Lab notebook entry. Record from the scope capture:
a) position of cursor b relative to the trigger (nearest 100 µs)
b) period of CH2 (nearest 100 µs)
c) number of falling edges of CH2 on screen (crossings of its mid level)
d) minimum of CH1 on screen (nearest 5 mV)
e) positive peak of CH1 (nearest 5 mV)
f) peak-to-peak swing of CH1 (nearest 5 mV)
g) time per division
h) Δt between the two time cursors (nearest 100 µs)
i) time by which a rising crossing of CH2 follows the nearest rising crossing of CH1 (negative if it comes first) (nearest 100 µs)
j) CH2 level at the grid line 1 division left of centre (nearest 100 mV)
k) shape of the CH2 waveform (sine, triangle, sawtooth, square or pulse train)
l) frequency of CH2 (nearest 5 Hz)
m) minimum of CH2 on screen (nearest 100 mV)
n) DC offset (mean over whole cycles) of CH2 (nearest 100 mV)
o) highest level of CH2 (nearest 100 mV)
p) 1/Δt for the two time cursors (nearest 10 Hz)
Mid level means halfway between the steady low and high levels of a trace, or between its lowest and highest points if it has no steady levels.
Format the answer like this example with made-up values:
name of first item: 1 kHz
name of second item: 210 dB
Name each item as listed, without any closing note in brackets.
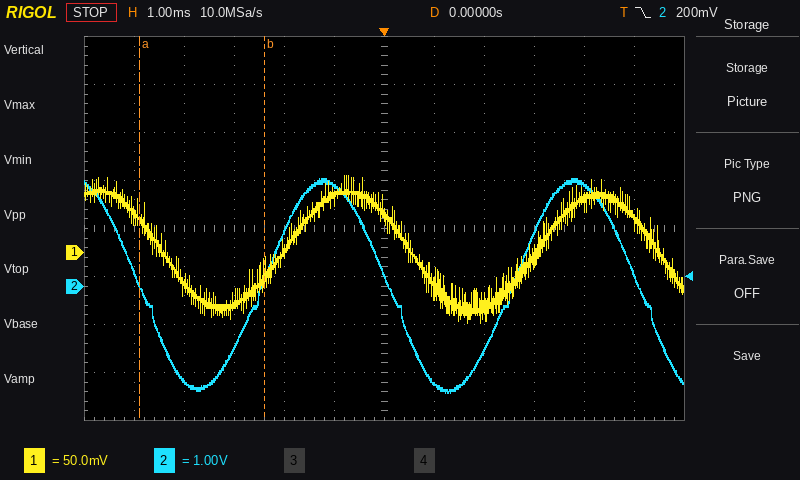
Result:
position of cursor b relative to the trigger: -2.4 ms
period of CH2: 5.0 ms
number of falling edges of CH2 on screen: 3
minimum of CH1 on screen: -75 mV
positive peak of CH1: 80 mV
peak-to-peak swing of CH1: 155 mV
time per division: 1 ms
Δt between the two time cursors: 2.5 ms
time by which a rising crossing of CH2 follows the nearest rising crossing of CH1 (negative if it comes first): -500 µs
CH2 level at the grid line 1 division left of centre: 2.1 V
shape of the CH2 waveform: sine
frequency of CH2: 200 Hz
minimum of CH2 on screen: -2.2 V
DC offset (mean over whole cycles) of CH2: 0.0 V
highest level of CH2: 2.2 V
1/Δt for the two time cursors: 400 Hz
